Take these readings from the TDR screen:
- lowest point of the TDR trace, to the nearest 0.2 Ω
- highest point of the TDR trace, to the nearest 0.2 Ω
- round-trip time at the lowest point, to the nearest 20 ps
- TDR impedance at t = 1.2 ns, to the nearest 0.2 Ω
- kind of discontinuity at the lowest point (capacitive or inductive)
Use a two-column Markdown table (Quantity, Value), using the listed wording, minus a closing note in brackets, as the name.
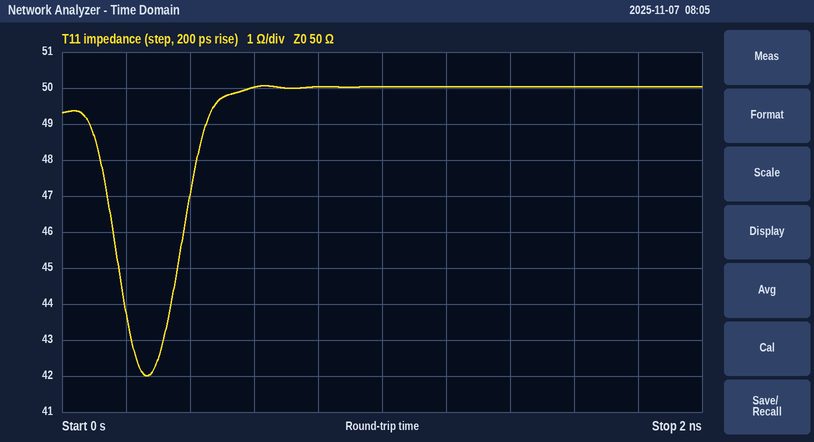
| Quantity | Value |
|---|---|
| lowest point of the TDR trace, to the nearest 0.2 Ω | 42.0 Ω |
| highest point of the TDR trace, to the nearest 0.2 Ω | 50.0 Ω |
| round-trip time at the lowest point, to the nearest 20 ps | 260 ps |
| TDR impedance at t = 1.2 ns, to the nearest 0.2 Ω | 50.0 Ω |
| kind of discontinuity at the lowest point | capacitive |
